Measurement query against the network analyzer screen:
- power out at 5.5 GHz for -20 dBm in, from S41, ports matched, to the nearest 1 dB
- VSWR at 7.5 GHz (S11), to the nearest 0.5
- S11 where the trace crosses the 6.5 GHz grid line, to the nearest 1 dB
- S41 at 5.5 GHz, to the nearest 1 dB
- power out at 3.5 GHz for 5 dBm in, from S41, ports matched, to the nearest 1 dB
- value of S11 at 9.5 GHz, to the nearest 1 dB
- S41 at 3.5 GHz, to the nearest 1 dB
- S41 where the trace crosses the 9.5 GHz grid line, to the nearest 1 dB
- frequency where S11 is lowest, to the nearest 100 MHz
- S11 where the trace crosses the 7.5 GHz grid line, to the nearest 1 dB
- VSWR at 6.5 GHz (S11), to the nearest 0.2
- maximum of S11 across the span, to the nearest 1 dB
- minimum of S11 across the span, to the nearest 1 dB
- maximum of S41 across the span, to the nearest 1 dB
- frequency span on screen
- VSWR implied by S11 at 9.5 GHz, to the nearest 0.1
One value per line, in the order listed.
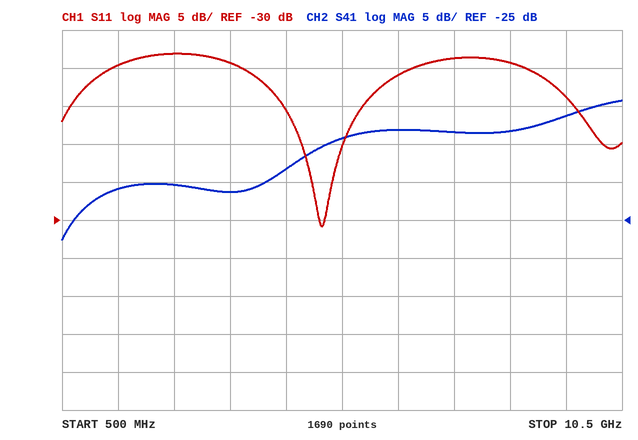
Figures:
-34 dBm
2.0
-11 dB
-14 dB
-16 dBm
-14 dB
-21 dB
-11 dB
5.1 GHz
-9 dB
1.8
-8 dB
-31 dB
-9 dB
10 GHz
1.5
